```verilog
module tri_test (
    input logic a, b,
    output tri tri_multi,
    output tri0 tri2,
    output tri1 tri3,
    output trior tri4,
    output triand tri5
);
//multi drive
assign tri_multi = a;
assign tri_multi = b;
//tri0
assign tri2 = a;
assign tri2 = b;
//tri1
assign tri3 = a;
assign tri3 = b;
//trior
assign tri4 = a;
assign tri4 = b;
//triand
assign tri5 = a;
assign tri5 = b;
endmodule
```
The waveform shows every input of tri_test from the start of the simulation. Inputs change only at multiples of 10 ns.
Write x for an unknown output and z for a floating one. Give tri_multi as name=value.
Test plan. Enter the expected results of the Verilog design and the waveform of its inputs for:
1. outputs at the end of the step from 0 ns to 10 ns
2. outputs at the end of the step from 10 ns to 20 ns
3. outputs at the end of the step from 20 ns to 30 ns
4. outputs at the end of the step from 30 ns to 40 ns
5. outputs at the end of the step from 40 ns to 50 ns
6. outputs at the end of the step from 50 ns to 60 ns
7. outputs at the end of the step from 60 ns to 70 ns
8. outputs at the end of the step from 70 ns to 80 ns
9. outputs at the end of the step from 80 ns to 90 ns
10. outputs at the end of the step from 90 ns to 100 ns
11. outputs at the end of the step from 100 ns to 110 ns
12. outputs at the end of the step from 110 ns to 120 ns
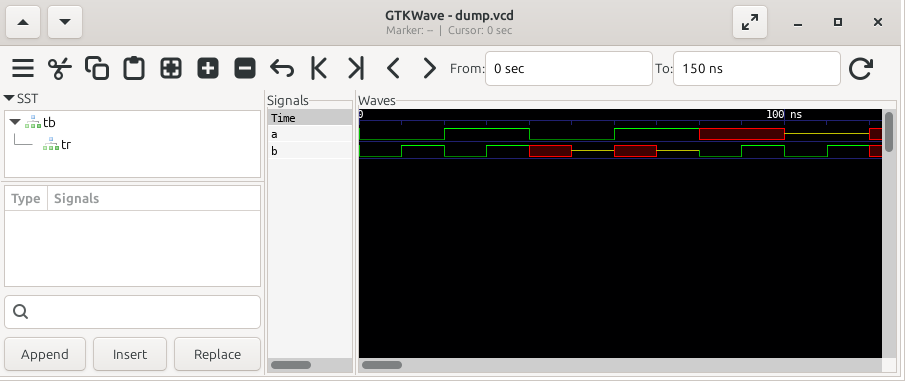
tri_multi=0
tri_multi=x
tri_multi=x
tri_multi=1
tri_multi=x
tri_multi=0
tri_multi=x
tri_multi=1
tri_multi=x
tri_multi=x
tri_multi=0
tri_multi=1
